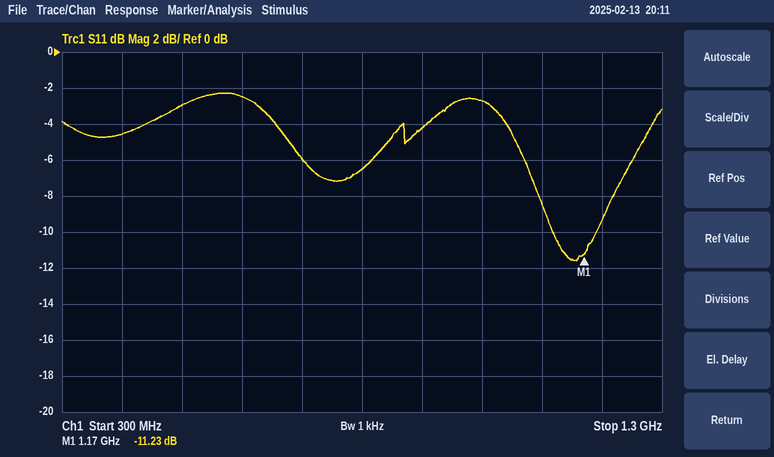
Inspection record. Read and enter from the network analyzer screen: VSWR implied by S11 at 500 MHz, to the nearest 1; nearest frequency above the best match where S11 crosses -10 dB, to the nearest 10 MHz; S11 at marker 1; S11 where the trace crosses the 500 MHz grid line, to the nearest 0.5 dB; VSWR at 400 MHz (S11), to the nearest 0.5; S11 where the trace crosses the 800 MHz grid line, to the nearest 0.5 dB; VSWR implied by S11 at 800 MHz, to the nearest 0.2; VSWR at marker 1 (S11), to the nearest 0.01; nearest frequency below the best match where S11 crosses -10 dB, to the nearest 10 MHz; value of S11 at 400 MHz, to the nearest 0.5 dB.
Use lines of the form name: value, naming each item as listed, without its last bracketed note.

VSWR implied by S11 at 500 MHz, to the nearest 1: 6
nearest frequency above the best match where S11 crosses -10 dB, to the nearest 10 MHz: 1.19 GHz
S11 at marker 1: -11.23 dB
S11 where the trace crosses the 500 MHz grid line, to the nearest 0.5 dB: -3.0 dB
VSWR at 400 MHz (S11), to the nearest 0.5: 4.0
S11 where the trace crosses the 800 MHz grid line, to the nearest 0.5 dB: -6.5 dB
VSWR implied by S11 at 800 MHz, to the nearest 0.2: 2.8
VSWR at marker 1 (S11), to the nearest 0.01: 1.76
nearest frequency below the best match where S11 crosses -10 dB, to the nearest 10 MHz: 1.12 GHz
value of S11 at 400 MHz, to the nearest 0.5 dB: -4.5 dB
